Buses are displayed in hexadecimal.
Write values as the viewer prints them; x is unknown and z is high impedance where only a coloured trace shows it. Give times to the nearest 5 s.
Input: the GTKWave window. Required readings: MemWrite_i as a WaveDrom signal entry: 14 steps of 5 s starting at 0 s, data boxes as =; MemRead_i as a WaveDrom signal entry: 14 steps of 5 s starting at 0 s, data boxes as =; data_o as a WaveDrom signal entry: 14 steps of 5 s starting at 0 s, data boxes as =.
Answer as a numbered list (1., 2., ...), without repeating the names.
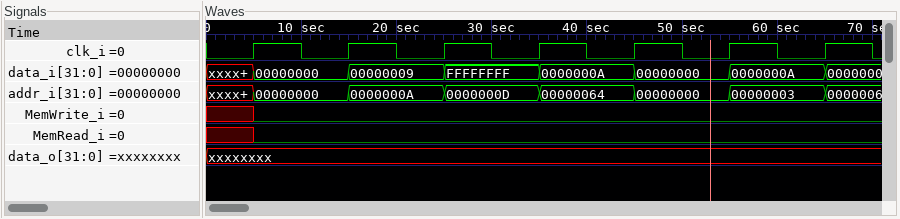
1. {name: 'MemWrite_i', wave: 'x0............'}
2. {name: 'MemRead_i', wave: 'x0............'}
3. {name: 'data_o', wave: 'x.............'}
